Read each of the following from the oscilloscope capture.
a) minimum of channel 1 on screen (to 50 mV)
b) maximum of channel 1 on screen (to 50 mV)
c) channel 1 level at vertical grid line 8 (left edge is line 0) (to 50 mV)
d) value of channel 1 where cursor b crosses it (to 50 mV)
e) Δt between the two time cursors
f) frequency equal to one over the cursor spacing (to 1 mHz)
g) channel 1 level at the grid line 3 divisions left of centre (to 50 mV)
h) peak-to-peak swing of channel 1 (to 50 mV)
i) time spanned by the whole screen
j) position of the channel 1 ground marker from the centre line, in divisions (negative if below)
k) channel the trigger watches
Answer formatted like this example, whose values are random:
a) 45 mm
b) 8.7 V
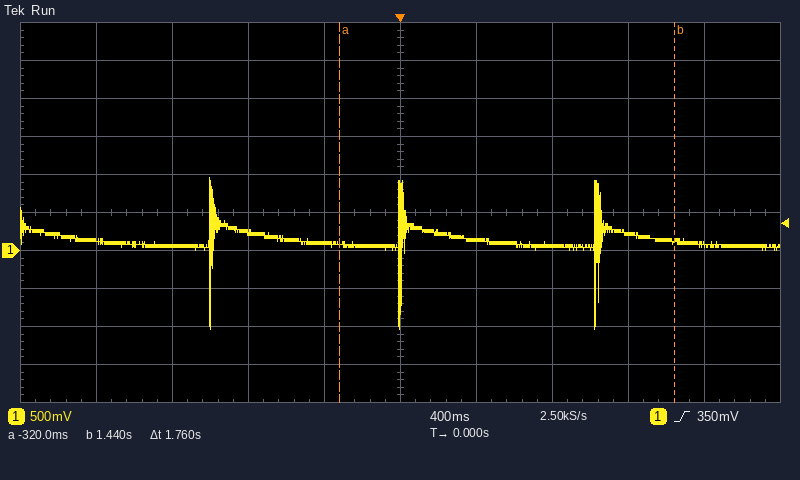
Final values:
a) -1.05 V
b) 950 mV
c) 200 mV
d) 100 mV
e) 1.76 s
f) 568 mHz
g) 50 mV
h) 2.00 V
i) 4 s
j) -1.0 div
k) channel 1
